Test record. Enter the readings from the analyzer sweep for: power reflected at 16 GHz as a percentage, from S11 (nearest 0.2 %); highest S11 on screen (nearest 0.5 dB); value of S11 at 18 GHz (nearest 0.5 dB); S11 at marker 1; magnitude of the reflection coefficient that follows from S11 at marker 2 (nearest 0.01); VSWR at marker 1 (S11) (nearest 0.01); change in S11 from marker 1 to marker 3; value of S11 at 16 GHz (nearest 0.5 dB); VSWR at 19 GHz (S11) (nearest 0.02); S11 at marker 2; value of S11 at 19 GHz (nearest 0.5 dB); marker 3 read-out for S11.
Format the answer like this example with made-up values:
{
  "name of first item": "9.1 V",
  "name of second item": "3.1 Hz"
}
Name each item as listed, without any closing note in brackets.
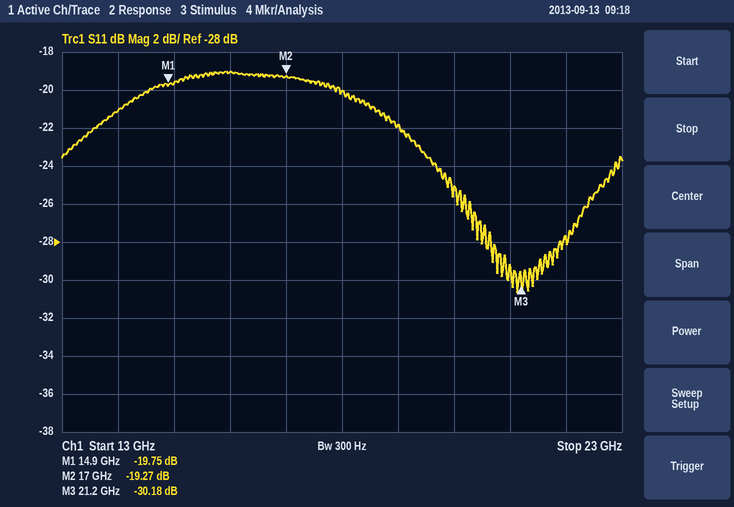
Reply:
{
  "power reflected at 16 GHz as a percentage, from S11": "1.2 %",
  "highest S11 on screen": "-19.0 dB",
  "value of S11 at 18 GHz": "-20.0 dB",
  "S11 at marker 1": "-19.75 dB",
  "magnitude of the reflection coefficient that follows from S11 at marker 2": "0.11",
  "VSWR at marker 1 (S11)": "1.23",
  "change in S11 from marker 1 to marker 3": "-10.43 dB",
  "value of S11 at 16 GHz": "-19.0 dB",
  "VSWR at 19 GHz (S11)": "1.18",
  "S11 at marker 2": "-19.27 dB",
  "value of S11 at 19 GHz": "-22.0 dB",
  "marker 3 read-out for S11": "-30.18 dB"
}
